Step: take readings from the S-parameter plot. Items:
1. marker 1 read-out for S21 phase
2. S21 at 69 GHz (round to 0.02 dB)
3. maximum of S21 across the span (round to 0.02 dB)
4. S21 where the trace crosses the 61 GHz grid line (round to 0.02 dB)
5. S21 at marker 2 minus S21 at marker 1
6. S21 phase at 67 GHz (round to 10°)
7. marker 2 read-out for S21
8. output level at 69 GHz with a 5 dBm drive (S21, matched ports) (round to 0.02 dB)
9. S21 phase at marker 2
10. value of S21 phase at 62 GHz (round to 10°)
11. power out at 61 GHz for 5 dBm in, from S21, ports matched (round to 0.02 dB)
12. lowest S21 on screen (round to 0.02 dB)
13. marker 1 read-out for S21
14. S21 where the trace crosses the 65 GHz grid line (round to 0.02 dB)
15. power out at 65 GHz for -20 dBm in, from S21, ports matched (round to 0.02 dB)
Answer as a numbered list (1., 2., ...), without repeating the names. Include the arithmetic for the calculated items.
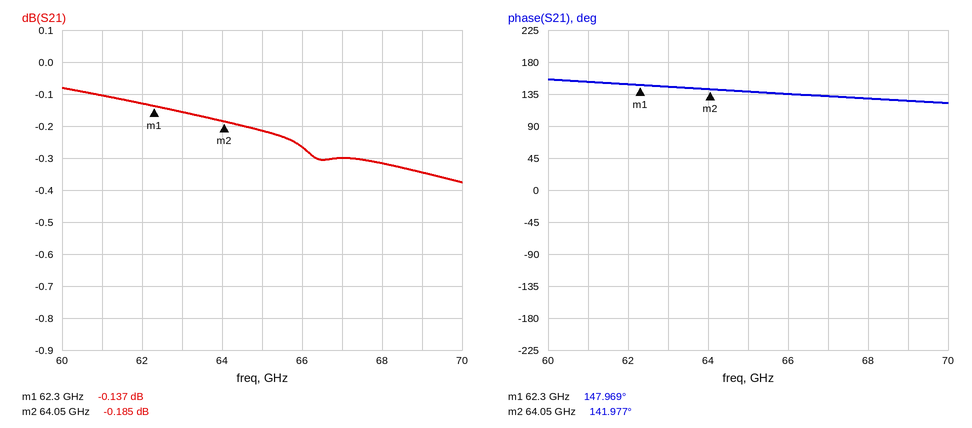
1. 147.969°
2. -0.34 dB
3. -0.08 dB
4. -0.10 dB
5. -0.185 − (-0.137) = -0.048 dB
6. 130°
7. -0.185 dB
8. 5 dBm + (-0.34 dB) = 4.66 dBm
9. 141.977°
10. 150°
11. 5 dBm + (-0.10 dB) = 4.90 dBm
12. -0.38 dB
13. -0.137 dB
14. -0.22 dB
15. -20 dBm + (-0.22 dB) = -20.22 dBm
